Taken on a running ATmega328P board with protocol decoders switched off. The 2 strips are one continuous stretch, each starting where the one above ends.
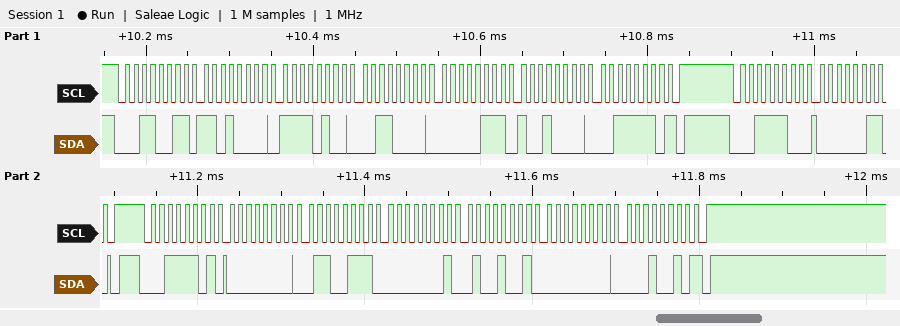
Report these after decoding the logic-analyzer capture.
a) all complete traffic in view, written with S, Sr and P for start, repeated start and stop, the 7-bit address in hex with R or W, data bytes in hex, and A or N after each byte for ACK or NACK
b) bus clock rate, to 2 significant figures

S 19R A D0 A F4 A 30 A 07 A 90 A 3E N P S 1EW A 03 A P S 1ER A 00 A 67 A 01 A 49 A 00 A 12 N P
100 kHz
